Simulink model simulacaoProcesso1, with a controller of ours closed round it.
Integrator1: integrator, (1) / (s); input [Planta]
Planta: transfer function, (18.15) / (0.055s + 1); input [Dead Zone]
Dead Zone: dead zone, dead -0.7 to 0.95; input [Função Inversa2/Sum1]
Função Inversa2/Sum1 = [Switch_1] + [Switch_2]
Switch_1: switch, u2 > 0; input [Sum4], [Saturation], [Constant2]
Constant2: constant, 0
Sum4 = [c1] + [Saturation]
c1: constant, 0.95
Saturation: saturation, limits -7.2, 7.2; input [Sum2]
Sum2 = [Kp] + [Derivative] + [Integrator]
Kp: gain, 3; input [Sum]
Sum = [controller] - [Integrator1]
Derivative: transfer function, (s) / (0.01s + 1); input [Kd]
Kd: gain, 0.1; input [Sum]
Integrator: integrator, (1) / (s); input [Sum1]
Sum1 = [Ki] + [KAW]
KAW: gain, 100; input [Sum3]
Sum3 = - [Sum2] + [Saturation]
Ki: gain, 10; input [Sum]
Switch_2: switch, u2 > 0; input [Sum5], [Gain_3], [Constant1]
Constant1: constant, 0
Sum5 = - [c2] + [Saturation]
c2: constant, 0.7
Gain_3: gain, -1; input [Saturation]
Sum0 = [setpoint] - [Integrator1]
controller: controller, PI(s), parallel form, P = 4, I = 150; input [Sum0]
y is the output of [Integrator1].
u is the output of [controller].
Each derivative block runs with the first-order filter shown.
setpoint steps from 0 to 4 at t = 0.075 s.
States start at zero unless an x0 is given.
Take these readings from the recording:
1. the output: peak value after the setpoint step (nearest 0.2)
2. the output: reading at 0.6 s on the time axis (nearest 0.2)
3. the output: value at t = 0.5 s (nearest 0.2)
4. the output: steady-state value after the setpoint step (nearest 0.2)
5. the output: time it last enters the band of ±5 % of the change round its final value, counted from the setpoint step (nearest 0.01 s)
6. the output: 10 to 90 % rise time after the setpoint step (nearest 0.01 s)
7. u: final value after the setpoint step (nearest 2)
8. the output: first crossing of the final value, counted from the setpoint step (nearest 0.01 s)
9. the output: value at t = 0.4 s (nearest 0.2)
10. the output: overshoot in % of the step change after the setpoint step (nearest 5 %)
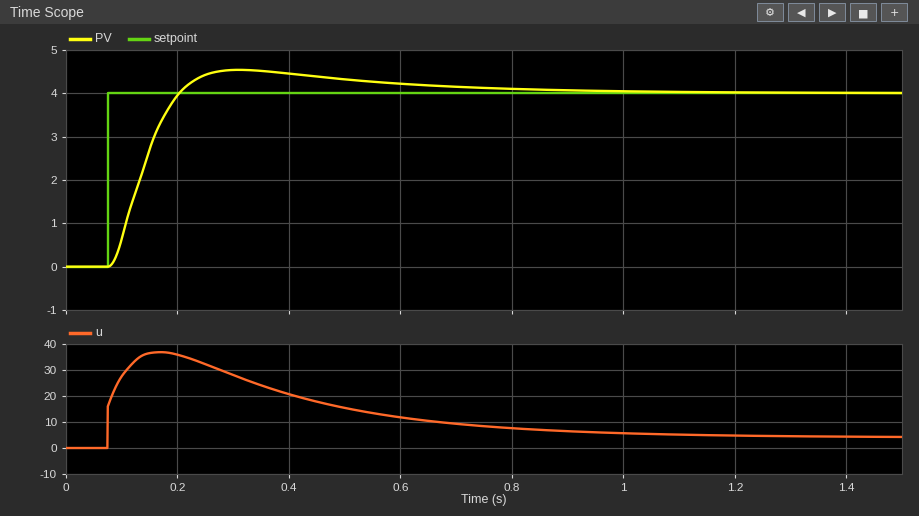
4.6
4.2
4.4
4.0
0.55 s
0.09 s
4
0.13 s
4.4
15 %
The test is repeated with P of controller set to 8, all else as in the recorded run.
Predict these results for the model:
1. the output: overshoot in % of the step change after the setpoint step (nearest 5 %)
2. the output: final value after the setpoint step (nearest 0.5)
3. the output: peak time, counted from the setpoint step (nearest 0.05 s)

20 %
4.0
0.30 s
